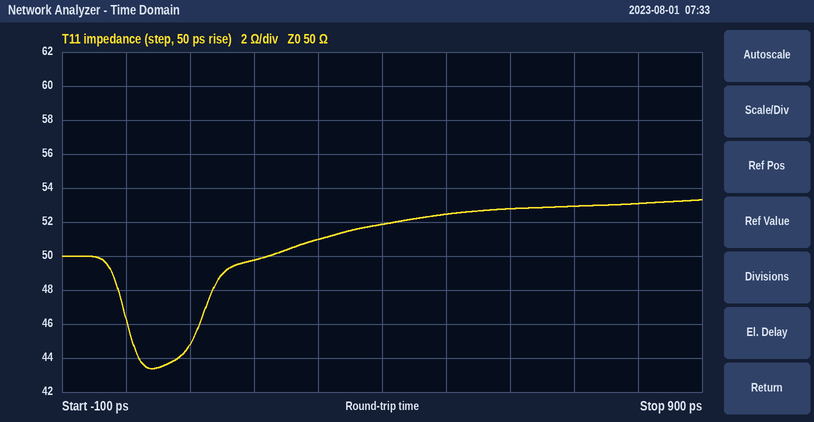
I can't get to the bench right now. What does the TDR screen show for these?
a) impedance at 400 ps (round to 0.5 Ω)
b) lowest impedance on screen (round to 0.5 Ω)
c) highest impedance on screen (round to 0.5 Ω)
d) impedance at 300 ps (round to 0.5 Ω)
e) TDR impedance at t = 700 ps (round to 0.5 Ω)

52.0 Ω
43.5 Ω
53.5 Ω
51.0 Ω
53.0 Ω
